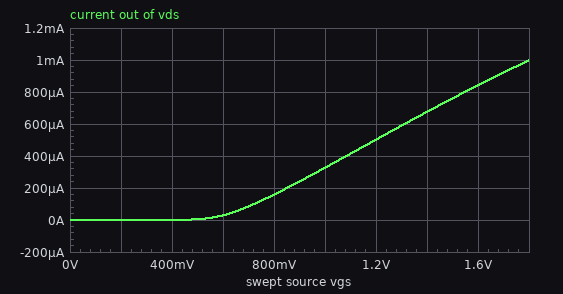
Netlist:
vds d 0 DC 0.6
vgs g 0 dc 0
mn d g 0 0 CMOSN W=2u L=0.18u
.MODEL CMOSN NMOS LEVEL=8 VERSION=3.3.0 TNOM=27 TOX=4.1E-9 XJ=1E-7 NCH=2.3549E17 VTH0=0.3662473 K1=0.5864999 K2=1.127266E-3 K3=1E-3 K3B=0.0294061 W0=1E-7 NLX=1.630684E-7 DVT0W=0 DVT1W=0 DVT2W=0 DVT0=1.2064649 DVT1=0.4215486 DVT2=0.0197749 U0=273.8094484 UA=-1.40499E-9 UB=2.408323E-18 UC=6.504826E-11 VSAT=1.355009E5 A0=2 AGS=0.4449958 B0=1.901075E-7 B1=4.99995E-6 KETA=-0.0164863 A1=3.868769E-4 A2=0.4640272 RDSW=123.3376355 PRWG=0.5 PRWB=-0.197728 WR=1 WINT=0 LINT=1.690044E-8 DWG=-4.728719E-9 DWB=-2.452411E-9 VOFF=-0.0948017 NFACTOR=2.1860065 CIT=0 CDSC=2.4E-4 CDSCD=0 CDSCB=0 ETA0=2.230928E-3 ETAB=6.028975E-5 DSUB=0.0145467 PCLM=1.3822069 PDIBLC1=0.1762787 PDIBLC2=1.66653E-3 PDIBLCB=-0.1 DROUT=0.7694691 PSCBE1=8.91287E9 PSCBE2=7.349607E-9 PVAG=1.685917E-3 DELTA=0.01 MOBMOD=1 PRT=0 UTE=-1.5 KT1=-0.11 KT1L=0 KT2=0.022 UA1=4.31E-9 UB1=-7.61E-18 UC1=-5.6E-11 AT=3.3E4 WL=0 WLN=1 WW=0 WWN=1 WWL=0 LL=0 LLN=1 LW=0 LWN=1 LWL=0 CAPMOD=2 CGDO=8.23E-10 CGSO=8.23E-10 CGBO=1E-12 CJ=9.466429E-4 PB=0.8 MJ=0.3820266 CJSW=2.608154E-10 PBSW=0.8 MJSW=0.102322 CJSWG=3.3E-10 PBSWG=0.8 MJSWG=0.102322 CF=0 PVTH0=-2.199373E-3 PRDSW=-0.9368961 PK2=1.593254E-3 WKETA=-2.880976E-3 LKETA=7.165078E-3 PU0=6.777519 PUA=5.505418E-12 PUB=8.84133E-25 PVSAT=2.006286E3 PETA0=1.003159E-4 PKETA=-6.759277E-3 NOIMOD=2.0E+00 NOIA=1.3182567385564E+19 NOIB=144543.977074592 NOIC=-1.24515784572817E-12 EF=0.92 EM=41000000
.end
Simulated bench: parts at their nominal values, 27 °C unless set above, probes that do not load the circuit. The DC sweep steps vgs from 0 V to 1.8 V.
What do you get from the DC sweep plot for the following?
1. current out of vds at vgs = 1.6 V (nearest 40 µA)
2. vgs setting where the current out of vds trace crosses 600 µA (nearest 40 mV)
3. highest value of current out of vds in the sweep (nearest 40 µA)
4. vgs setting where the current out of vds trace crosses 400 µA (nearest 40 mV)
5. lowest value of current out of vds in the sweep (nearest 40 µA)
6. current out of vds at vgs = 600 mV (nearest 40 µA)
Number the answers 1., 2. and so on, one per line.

1. 840 µA
2. 1.32 V
3. 1.00 mA
4. 1.08 V
5. 0 A
6. 40 µA
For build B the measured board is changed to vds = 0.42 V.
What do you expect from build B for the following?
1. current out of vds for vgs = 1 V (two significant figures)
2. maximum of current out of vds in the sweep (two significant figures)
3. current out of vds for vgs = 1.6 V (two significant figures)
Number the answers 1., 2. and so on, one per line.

1. 310 µA
2. 890 µA
3. 770 µA
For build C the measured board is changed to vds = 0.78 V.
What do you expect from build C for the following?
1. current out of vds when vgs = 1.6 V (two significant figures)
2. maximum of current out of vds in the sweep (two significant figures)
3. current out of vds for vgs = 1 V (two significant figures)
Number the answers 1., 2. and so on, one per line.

1. 870 µA
2. 1.0 mA
3. 340 µA
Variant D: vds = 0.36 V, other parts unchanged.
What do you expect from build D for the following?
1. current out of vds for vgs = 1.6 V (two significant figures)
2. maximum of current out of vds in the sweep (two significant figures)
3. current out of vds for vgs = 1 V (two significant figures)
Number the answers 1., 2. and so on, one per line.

1. 720 µA
2. 810 µA
3. 300 µA
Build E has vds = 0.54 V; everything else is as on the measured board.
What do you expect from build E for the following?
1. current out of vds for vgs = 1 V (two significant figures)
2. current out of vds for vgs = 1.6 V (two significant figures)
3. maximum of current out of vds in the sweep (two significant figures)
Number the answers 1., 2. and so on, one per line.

1. 320 µA
2. 830 µA
3. 970 µA
